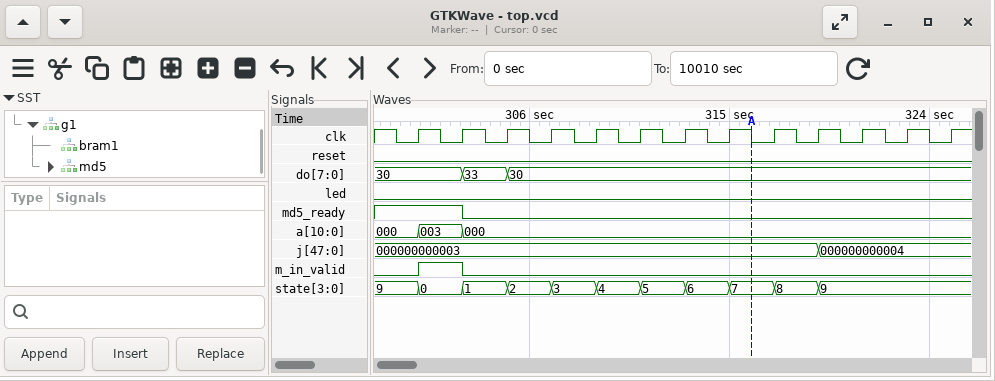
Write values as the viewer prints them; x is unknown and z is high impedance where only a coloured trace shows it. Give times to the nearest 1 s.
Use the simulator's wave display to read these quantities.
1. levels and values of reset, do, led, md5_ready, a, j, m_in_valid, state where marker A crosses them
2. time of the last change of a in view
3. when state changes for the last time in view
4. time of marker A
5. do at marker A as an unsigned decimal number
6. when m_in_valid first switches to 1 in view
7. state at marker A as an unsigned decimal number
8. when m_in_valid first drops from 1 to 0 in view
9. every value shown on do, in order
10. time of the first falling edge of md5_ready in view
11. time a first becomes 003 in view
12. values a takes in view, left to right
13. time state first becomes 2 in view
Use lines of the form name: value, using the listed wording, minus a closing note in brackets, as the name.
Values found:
levels and values of reset, do, led, md5_ready, a, j, m_in_valid, state where marker A crosses them: reset=0, do=30, led=0, md5_ready=0, a=000, j=000000000003, m_in_valid=0, state=7
time of the last change of a in view: 303 s
when state changes for the last time in view: 319 s
time of marker A: 316 s
do at marker A as an unsigned decimal number: 48
when m_in_valid first switches to 1 in view: 301 s
state at marker A as an unsigned decimal number: 7
when m_in_valid first drops from 1 to 0 in view: 303 s
every value shown on do, in order: 30, 33, 30
time of the first falling edge of md5_ready in view: 303 s
time a first becomes 003 in view: 301 s
values a takes in view, left to right: 000, 003, 000
time state first becomes 2 in view: 305 s
